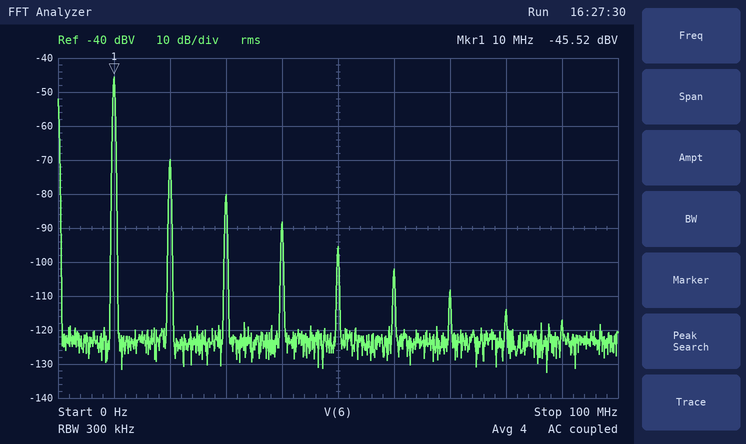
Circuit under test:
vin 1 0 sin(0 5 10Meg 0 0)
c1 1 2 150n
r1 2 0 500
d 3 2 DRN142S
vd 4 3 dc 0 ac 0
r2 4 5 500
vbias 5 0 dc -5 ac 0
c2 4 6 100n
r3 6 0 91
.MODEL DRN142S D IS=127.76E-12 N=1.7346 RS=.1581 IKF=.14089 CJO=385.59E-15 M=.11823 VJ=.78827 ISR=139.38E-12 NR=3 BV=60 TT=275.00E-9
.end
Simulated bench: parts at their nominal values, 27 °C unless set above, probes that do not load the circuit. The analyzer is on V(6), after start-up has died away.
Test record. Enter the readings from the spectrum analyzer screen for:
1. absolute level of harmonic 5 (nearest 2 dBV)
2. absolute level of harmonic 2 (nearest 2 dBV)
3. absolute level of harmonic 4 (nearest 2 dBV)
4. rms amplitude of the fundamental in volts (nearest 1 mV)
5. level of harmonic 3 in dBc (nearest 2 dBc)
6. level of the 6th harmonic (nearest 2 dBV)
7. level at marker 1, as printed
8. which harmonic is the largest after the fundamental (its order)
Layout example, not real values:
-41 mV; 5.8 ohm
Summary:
-96 dBV; -70 dBV; -88 dBV; 5 mV; -34 dBc; -102 dBV; -45.52 dBV; 2
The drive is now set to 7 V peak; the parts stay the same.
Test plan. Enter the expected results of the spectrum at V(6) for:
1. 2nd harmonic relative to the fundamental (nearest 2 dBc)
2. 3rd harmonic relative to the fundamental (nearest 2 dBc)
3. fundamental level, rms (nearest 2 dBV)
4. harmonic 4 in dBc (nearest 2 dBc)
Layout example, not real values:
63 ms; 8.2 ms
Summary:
4 dBc; 4 dBc; -12 dBV; 0 dBc
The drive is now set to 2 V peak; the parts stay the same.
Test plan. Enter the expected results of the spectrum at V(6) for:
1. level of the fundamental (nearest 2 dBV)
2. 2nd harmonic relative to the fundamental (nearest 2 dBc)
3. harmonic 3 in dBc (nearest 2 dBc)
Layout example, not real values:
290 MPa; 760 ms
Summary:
-54 dBV; -34 dBc; -54 dBc
